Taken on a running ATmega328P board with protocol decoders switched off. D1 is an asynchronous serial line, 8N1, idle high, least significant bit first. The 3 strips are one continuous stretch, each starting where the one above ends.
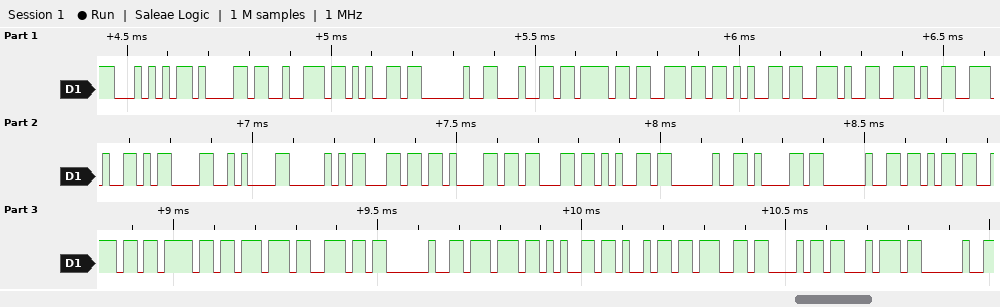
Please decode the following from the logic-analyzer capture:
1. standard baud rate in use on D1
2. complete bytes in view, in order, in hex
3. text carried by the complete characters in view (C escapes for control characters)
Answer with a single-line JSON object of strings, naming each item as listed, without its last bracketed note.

{"standard baud rate in use on D1": "57600 baud", "complete bytes in view, in order, in hex": "54 61 72 65 20 64 6F 6E 65 2E 2E 2E 0D 0A 50 6C 61 63 65 20 61 20 6B 6E 6F 77 6E 20 77 65 69 67 68 74 20", "text carried by the complete characters in view": "\"Tare done...\\r\\nPlace a known weight \""}
